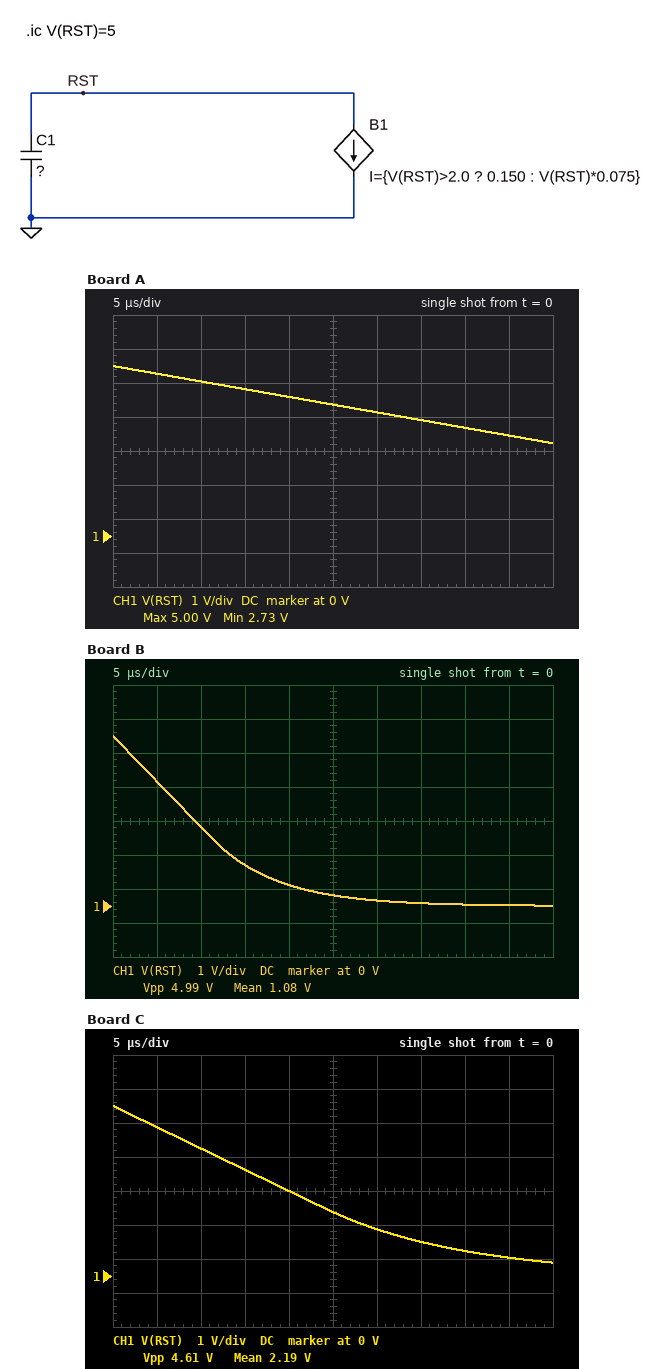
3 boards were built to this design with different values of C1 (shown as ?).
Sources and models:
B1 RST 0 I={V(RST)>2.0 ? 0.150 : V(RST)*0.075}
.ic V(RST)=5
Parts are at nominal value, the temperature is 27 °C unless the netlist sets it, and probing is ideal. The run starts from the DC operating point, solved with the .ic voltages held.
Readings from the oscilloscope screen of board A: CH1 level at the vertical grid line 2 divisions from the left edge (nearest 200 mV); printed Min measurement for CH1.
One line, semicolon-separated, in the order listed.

4.6 V; 2.73 V
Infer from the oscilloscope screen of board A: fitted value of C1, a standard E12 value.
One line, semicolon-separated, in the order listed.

3.3 µF
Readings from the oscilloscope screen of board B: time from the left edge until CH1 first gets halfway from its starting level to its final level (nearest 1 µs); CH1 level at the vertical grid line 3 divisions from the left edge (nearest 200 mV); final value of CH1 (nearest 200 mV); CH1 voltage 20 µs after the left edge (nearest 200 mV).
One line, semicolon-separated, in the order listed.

9 µs; 1.2 V; 0 V; 600 mV
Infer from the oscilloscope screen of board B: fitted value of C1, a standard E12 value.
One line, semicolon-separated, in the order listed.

560 nF
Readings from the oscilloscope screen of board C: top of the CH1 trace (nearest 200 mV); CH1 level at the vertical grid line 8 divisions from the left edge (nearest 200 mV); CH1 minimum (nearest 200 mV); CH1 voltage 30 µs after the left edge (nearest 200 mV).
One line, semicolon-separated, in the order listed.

5.0 V; 800 mV; 400 mV; 1.4 V
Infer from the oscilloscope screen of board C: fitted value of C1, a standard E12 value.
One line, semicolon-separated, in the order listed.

1.2 µF
